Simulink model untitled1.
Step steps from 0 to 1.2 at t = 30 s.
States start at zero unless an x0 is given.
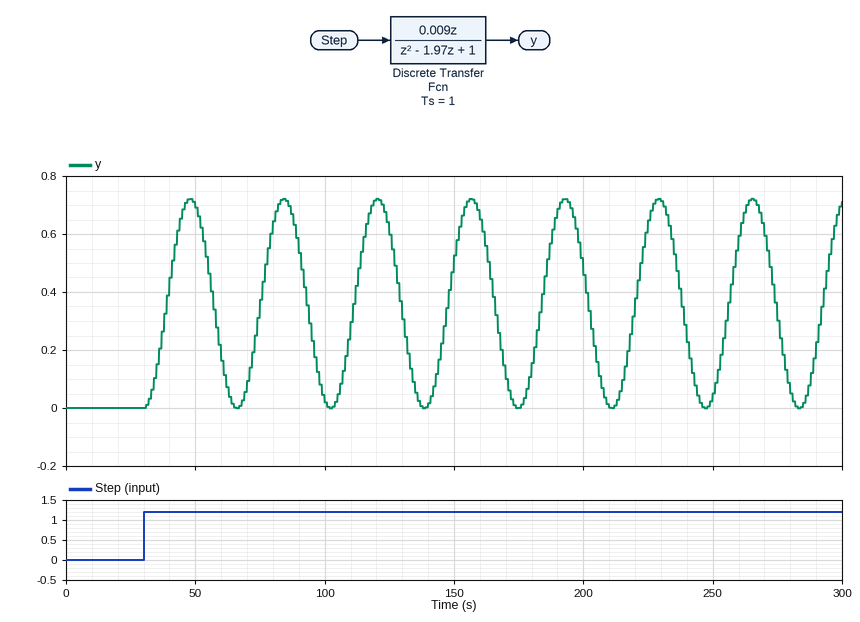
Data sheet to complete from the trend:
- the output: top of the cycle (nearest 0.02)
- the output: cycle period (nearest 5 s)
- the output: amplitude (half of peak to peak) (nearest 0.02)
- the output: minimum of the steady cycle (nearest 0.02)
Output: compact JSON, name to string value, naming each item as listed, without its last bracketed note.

{"the output: top of the cycle": "0.72", "the output: cycle period": "35 s", "the output: amplitude (half of peak to peak)": "0.36", "the output: minimum of the steady cycle": "0.00"}
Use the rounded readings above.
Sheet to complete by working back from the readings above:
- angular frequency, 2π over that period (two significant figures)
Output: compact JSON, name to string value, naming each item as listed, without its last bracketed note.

{"angular frequency, 2π over that period": "0.18 rad/s"}
